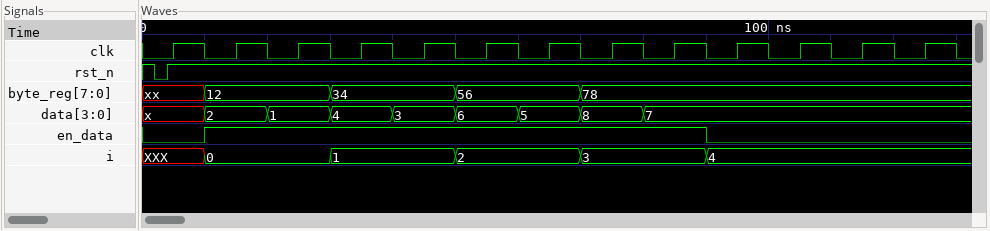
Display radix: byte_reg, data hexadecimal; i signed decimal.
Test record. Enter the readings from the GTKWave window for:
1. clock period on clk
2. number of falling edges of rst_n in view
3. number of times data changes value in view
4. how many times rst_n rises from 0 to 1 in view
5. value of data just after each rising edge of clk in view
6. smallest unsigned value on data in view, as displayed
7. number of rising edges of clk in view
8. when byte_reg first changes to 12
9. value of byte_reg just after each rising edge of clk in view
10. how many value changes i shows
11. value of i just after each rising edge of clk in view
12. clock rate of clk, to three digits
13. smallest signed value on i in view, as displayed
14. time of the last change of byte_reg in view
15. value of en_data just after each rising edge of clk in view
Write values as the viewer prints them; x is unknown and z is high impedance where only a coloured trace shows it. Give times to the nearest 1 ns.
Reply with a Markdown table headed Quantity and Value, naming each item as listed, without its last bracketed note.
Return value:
| Quantity | Value |
|---|---|
| clock period on clk | 10 ns |
| number of falling edges of rst_n in view | 1 |
| number of times data changes value in view | 8 |
| how many times rst_n rises from 0 to 1 in view | 1 |
| value of data just after each rising edge of clk in view | x, 2, 1, 4, 3, 6, 5, 8, 7, 7, 7, 7, 7 |
| smallest unsigned value on data in view, as displayed | 1 |
| number of rising edges of clk in view | 13 |
| when byte_reg first changes to 12 | 10 ns |
| value of byte_reg just after each rising edge of clk in view | xx, 12, 12, 34, 34, 56, 56, 78, 78, 78, 78, 78, 78 |
| how many value changes i shows | 5 |
| value of i just after each rising edge of clk in view | XXX, 0, 0, 1, 1, 2, 2, 3, 3, 4, 4, 4, 4 |
| clock rate of clk, to three digits | 100 MHz |
| smallest signed value on i in view, as displayed | 0 |
| time of the last change of byte_reg in view | 70 ns |
| value of en_data just after each rising edge of clk in view | 0 1 1 1 1 1 1 1 1 0 0 0 0 |
